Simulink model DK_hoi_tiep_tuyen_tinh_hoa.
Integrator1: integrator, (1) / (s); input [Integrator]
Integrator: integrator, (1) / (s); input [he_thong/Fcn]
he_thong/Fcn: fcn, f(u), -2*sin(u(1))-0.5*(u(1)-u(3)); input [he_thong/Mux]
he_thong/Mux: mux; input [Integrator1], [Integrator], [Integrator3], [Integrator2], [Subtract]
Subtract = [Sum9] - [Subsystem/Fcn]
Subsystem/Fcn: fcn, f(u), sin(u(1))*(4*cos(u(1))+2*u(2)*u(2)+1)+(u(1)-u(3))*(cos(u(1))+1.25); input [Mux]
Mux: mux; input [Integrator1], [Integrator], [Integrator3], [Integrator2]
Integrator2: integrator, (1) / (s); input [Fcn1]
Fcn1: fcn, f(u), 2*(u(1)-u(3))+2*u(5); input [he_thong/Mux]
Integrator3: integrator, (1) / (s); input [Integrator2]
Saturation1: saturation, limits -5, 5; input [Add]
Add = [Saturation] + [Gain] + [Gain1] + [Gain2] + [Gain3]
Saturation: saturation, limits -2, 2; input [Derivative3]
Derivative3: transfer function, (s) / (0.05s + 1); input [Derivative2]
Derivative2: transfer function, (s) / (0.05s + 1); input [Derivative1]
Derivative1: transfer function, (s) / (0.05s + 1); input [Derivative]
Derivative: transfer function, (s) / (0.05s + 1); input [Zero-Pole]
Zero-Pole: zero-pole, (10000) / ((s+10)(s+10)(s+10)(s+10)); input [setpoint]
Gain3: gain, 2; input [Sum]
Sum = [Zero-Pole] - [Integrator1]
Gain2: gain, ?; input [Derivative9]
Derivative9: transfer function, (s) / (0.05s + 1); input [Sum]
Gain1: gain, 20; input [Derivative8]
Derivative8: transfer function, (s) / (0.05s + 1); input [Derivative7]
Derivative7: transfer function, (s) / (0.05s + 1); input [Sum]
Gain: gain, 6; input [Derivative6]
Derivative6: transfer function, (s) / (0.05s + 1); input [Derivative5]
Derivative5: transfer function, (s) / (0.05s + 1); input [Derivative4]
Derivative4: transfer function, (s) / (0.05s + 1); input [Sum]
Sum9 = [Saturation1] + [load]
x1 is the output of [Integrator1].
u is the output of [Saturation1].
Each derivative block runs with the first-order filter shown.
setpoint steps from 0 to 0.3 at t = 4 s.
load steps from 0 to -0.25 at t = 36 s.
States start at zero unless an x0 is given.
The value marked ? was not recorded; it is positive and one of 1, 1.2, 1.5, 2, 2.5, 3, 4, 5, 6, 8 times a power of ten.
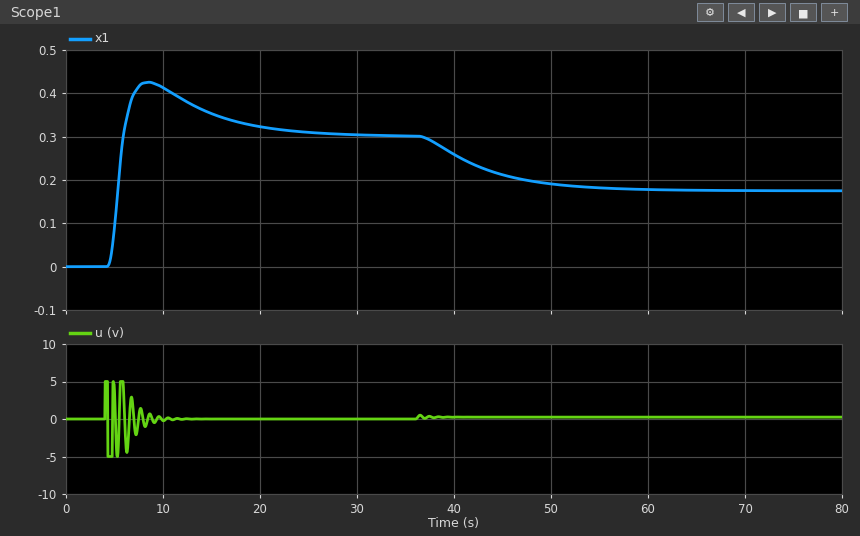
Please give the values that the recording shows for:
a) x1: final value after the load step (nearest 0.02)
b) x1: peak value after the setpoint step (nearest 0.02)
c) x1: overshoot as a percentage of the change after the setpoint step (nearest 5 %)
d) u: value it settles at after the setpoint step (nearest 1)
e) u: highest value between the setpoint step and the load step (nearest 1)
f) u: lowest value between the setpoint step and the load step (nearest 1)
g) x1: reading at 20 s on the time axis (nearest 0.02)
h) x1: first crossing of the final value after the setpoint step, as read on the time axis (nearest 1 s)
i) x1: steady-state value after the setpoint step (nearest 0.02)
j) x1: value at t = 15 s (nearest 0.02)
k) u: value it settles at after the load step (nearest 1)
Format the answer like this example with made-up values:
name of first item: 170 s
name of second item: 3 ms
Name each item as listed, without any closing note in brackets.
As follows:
x1: final value after the load step: 0.18
x1: peak value after the setpoint step: 0.42
x1: overshoot as a percentage of the change after the setpoint step: 40 %
u: value it settles at after the setpoint step: 0
u: highest value between the setpoint step and the load step: 5
u: lowest value between the setpoint step and the load step: -5
x1: reading at 20 s on the time axis: 0.32
x1: first crossing of the final value after the setpoint step, as read on the time axis: 6 s
x1: steady-state value after the setpoint step: 0.30
x1: value at t = 15 s: 0.36
u: value it settles at after the load step: 0
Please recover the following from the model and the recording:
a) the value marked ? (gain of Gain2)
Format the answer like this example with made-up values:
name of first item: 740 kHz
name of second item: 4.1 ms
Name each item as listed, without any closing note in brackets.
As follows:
the value marked ?: 15
